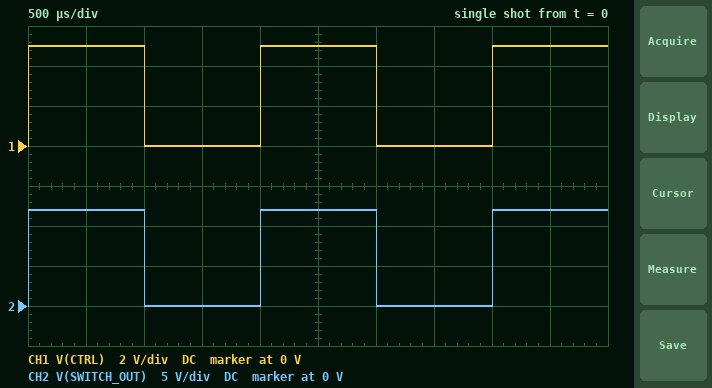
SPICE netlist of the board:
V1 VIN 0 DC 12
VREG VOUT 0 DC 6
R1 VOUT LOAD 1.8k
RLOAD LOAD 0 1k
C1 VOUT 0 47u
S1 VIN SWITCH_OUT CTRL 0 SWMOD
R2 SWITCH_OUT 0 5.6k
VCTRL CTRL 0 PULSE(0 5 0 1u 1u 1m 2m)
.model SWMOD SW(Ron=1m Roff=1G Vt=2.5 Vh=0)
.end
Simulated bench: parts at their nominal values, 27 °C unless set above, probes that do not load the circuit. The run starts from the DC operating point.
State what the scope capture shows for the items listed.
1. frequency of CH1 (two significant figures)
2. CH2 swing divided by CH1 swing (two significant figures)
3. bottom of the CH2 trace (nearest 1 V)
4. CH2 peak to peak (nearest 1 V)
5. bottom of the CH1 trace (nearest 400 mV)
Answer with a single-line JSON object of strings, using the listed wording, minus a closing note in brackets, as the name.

{"frequency of CH1": "500 Hz", "CH2 swing divided by CH1 swing": "2.4", "bottom of the CH2 trace": "0 V", "CH2 peak to peak": "12 V", "bottom of the CH1 trace": "0 V"}
